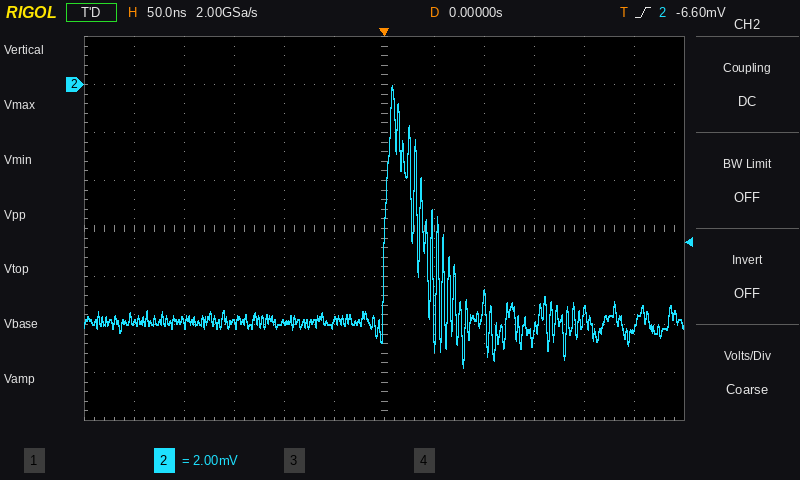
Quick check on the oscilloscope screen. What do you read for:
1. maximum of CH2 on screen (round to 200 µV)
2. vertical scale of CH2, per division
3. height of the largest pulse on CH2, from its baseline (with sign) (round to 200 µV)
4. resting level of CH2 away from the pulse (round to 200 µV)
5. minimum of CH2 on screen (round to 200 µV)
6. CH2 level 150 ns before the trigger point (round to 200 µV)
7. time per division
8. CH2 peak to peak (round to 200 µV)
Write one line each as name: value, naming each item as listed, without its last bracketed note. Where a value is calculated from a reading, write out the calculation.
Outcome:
maximum of CH2 on screen: 0.0 mV
vertical scale of CH2, per division: 2 mV
height of the largest pulse on CH2, from its baseline (with sign): 0.0 mV − (-9.8 mV) = +9.8 mV
resting level of CH2 away from the pulse: -9.8 mV
minimum of CH2 on screen: -11.8 mV
CH2 level 150 ns before the trigger point: -10.0 mV
time per division: 50 ns
CH2 peak to peak: 0.0 mV − (-11.8 mV) = 11.8 mV
